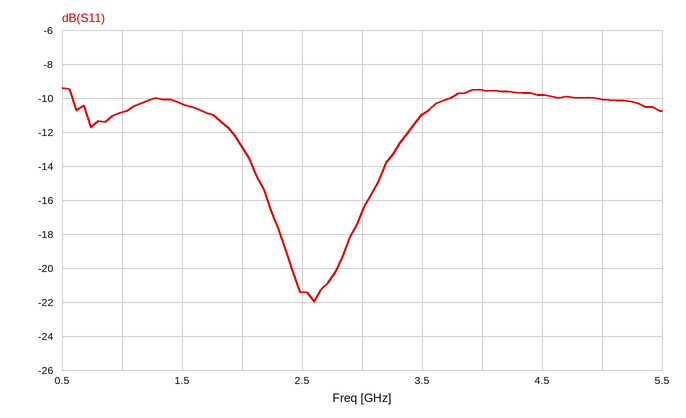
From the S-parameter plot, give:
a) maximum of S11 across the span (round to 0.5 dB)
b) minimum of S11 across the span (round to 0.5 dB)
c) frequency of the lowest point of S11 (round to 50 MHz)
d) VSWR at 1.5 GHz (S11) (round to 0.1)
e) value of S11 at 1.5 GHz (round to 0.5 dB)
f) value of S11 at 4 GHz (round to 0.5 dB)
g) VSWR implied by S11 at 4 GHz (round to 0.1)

-9.5 dB
-22.0 dB
2.60 GHz
1.9
-10.5 dB
-9.5 dB
2.0
